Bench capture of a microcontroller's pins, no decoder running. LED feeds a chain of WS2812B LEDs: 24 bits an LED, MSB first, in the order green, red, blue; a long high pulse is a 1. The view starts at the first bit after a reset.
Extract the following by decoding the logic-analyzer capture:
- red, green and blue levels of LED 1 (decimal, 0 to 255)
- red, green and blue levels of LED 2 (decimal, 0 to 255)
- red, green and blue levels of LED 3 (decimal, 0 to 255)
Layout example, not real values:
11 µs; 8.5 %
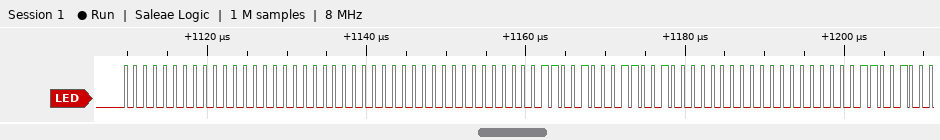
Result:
0, 0, 0; 0, 0, 50; 0, 50, 0
